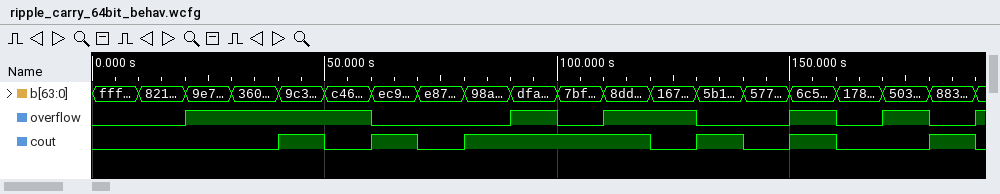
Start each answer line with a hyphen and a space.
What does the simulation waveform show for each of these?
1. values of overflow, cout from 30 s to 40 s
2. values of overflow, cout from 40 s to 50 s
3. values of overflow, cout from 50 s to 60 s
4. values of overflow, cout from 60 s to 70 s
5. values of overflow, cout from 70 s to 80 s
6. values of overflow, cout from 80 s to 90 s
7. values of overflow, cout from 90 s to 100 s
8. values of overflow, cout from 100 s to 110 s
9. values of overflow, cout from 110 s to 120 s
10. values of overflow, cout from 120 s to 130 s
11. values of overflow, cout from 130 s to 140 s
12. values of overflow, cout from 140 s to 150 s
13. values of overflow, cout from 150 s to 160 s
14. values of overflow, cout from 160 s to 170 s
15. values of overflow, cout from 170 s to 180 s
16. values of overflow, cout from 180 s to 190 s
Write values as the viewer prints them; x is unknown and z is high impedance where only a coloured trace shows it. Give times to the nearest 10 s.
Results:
- overflow=1, cout=0
- overflow=1, cout=1
- overflow=1, cout=0
- overflow=0, cout=1
- overflow=0, cout=0
- overflow=0, cout=1
- overflow=1, cout=1
- overflow=0, cout=1
- overflow=1, cout=1
- overflow=1, cout=0
- overflow=0, cout=1
- overflow=0, cout=0
- overflow=1, cout=1
- overflow=0, cout=0
- overflow=1, cout=0
- overflow=0, cout=1
